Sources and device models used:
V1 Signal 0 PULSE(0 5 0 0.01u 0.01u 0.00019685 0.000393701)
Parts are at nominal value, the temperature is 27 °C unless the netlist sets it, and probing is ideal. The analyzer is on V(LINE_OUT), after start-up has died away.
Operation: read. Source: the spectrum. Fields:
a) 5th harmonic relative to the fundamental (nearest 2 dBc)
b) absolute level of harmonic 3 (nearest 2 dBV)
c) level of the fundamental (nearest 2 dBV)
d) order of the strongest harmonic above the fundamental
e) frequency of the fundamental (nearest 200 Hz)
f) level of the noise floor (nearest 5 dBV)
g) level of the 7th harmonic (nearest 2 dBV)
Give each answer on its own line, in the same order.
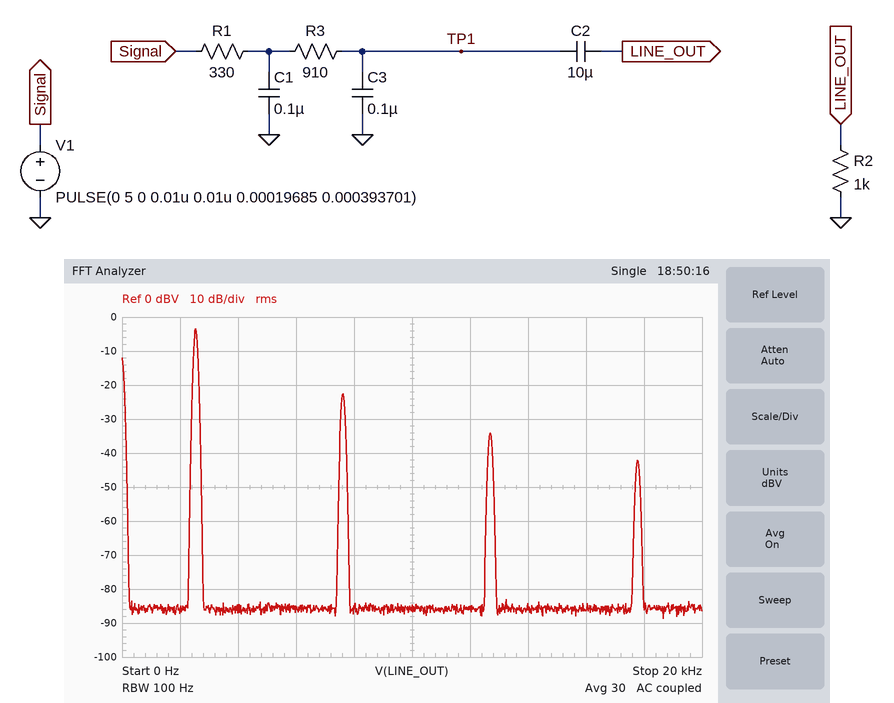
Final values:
-30 dBc
-22 dBV
-4 dBV
3
2.6 kHz
-85 dBV
-42 dBV
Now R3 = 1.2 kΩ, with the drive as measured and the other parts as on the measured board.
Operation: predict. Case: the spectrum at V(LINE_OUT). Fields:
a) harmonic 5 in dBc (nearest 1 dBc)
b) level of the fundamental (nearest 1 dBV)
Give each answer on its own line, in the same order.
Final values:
-31 dBc
-5 dBV
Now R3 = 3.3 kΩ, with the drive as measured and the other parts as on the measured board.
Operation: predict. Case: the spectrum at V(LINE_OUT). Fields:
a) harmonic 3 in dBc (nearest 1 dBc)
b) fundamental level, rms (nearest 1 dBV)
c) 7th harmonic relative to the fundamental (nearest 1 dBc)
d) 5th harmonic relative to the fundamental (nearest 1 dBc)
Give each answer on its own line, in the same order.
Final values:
-21 dBc
-11 dBV
-42 dBc
-33 dBc
